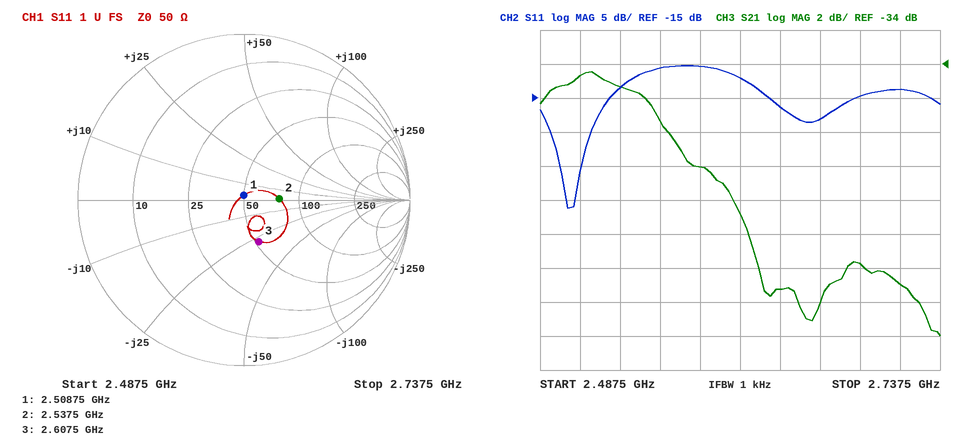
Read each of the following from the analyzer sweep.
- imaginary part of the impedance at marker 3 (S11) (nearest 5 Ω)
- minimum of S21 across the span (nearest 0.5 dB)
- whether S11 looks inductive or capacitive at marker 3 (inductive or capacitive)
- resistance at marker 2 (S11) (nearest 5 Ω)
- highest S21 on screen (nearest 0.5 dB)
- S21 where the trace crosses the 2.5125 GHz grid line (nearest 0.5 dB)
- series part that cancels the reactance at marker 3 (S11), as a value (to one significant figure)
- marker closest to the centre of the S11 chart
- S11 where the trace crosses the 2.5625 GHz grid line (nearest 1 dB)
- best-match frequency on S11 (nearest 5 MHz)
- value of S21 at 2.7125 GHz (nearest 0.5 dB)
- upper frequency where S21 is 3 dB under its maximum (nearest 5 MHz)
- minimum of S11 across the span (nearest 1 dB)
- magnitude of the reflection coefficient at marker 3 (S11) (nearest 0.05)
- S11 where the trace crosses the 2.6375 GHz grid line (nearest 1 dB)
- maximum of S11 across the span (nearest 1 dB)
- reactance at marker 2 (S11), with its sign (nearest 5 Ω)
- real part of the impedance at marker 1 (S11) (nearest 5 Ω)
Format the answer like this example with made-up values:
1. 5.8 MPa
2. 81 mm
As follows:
1. -30 Ω
2. -50.0 dB
3. capacitive
4. 75 Ω
5. -34.5 dB
6. -34.5 dB
7. 2 nH
8. marker 1
9. -11 dB
10. 2.505 GHz
11. -47.0 dB
12. 2.565 GHz
13. -31 dB
14. 0.25
15. -16 dB
16. -10 dB
17. 0 Ω
18. 50 Ω
